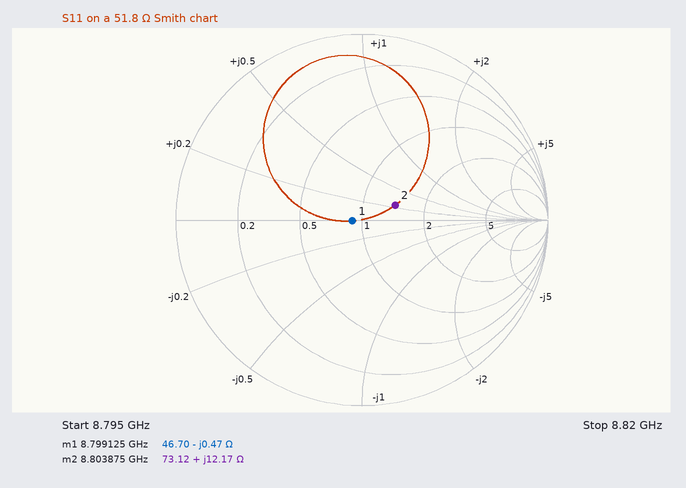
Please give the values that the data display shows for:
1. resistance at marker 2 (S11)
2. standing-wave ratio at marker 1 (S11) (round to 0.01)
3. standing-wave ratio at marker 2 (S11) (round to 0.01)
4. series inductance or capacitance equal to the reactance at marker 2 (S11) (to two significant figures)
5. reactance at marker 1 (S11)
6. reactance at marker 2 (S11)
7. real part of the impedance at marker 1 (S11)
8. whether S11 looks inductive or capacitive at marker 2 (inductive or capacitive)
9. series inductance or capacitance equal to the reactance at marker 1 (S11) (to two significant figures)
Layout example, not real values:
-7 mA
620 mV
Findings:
73.12 Ω
1.11
1.49
220 pH
-0.47 Ω
+12.17 Ω
46.70 Ω
inductive
38 pF
